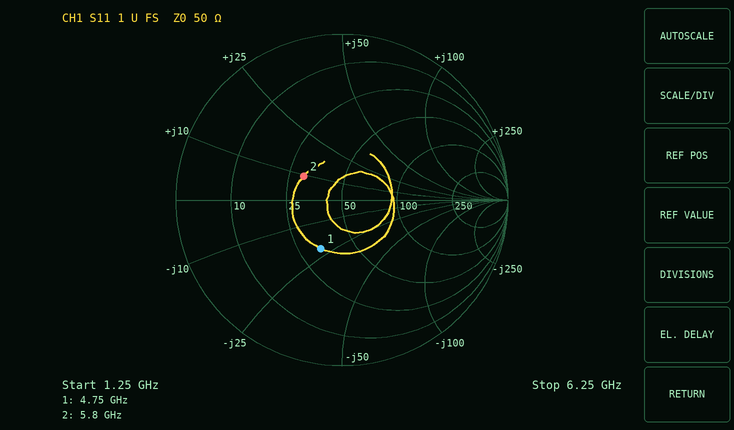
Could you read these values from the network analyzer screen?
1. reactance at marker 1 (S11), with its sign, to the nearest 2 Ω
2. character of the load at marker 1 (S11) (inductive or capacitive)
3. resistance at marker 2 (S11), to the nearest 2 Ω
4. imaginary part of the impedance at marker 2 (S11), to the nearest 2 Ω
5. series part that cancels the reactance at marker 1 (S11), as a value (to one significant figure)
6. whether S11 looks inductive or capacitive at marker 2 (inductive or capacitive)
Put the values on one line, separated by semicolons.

-22 Ω; capacitive; 30 Ω; +10 Ω; 700 pH; inductive
